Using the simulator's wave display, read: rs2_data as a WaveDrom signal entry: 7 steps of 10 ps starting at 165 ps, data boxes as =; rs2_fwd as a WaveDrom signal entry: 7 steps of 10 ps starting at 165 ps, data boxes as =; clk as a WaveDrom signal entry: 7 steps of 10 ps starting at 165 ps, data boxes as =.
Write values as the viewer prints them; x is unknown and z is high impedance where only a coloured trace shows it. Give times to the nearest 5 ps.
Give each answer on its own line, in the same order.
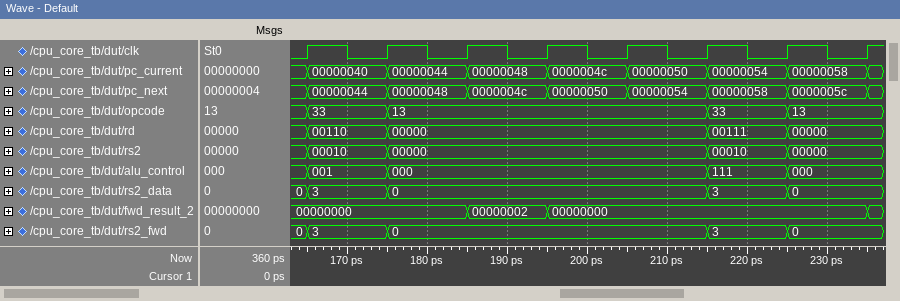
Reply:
{name: 'rs2_data', wave: '==...==', data: '3 0 3 0'}
{name: 'rs2_fwd', wave: '==...==', data: '3 0 3 0'}
{name: 'clk', wave: 'p......'}
